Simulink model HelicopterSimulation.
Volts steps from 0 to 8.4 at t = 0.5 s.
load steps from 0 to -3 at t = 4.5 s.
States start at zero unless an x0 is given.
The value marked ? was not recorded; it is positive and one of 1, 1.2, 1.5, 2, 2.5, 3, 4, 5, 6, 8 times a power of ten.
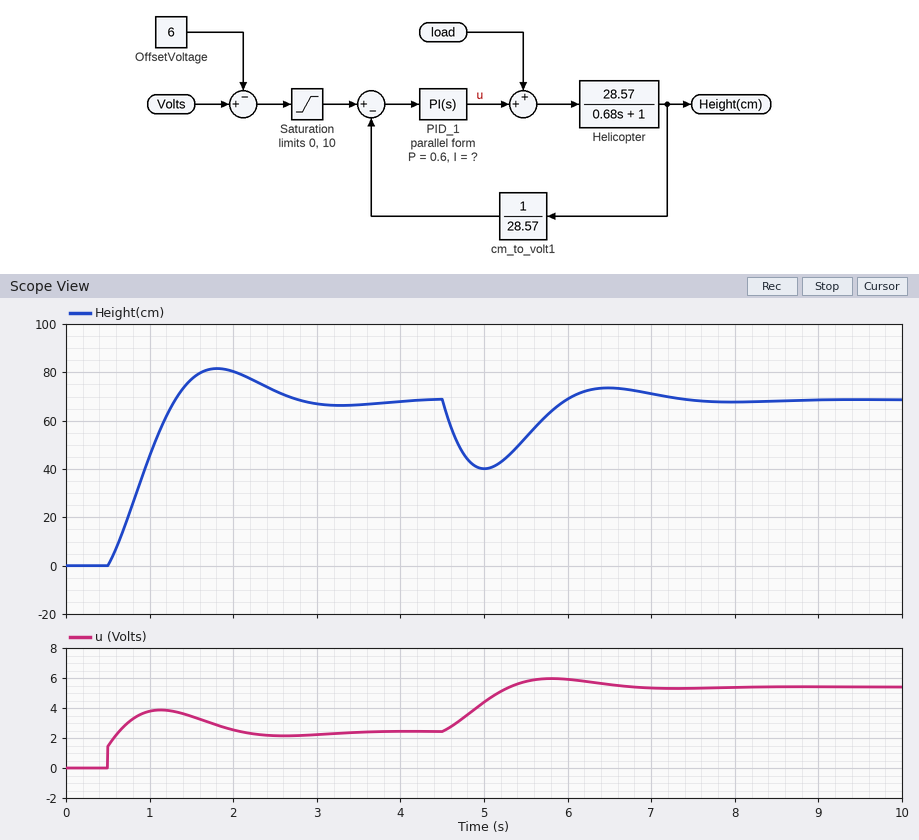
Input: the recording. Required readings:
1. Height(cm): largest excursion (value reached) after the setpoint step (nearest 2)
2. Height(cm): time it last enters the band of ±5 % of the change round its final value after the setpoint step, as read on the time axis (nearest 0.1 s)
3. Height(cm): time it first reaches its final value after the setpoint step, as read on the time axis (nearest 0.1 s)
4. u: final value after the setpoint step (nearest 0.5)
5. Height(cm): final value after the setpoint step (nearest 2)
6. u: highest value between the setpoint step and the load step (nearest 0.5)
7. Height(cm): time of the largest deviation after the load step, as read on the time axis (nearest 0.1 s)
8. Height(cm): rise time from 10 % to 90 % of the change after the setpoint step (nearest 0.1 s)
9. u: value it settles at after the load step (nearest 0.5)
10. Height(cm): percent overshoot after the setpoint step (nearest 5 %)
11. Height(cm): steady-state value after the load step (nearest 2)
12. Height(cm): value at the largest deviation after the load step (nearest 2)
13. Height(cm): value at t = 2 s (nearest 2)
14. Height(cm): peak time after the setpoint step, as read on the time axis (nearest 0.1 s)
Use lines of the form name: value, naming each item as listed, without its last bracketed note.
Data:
Height(cm): largest excursion (value reached) after the setpoint step: 82
Height(cm): time it last enters the band of ±5 % of the change round its final value after the setpoint step, as read on the time axis: 2.5 s
Height(cm): time it first reaches its final value after the setpoint step, as read on the time axis: 1.3 s
u: final value after the setpoint step: 2.5
Height(cm): final value after the setpoint step: 68
u: highest value between the setpoint step and the load step: 4.0
Height(cm): time of the largest deviation after the load step, as read on the time axis: 5.0 s
Height(cm): rise time from 10 % to 90 % of the change after the setpoint step: 0.6 s
u: value it settles at after the load step: 5.5
Height(cm): percent overshoot after the setpoint step: 20 %
Height(cm): steady-state value after the load step: 68
Height(cm): value at the largest deviation after the load step: 40
Height(cm): value at t = 2 s: 80
Height(cm): peak time after the setpoint step, as read on the time axis: 1.8 s
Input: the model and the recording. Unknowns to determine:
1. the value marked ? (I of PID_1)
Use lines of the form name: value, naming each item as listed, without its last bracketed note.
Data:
the value marked ?: 4
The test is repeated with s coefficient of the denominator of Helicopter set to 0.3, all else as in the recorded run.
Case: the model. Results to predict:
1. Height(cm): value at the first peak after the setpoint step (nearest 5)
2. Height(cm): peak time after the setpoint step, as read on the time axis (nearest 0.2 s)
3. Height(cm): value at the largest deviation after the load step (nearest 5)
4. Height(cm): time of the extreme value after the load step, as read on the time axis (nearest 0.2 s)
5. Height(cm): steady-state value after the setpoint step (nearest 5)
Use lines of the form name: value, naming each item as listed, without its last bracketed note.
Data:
Height(cm): value at the first peak after the setpoint step: 70
Height(cm): peak time after the setpoint step, as read on the time axis: 1.6 s
Height(cm): value at the largest deviation after the load step: 35
Height(cm): time of the extreme value after the load step, as read on the time axis: 4.8 s
Height(cm): steady-state value after the setpoint step: 70
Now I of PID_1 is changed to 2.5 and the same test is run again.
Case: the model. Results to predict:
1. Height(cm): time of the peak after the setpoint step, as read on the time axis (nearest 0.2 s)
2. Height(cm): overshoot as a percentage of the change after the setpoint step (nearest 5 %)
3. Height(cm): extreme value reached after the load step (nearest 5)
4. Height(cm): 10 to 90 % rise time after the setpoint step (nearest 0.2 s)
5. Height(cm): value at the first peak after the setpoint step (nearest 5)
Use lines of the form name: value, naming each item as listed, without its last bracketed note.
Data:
Height(cm): time of the peak after the setpoint step, as read on the time axis: 2.2 s
Height(cm): overshoot as a percentage of the change after the setpoint step: 10 %
Height(cm): extreme value reached after the load step: 35
Height(cm): 10 to 90 % rise time after the setpoint step: 0.8 s
Height(cm): value at the first peak after the setpoint step: 75
